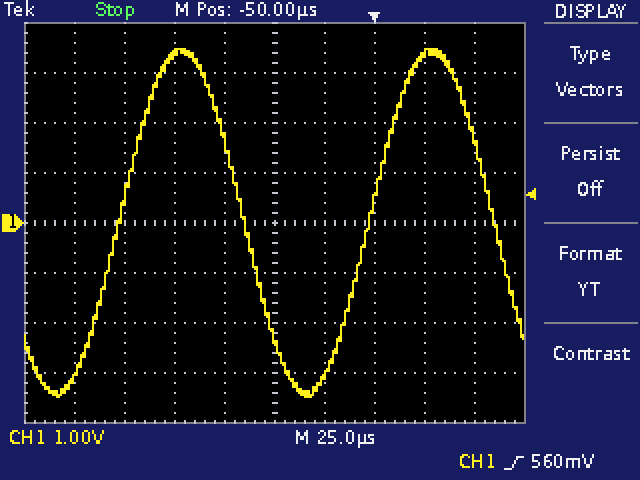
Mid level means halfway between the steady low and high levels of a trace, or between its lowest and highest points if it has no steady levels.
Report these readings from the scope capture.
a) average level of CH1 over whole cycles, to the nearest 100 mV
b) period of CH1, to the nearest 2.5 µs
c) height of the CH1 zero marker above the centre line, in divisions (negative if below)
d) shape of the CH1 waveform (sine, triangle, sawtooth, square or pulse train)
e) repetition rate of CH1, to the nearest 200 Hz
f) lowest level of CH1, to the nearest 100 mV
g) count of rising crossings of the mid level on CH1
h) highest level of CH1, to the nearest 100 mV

0.0 V
125.0 µs
0.0 div
sine
8.0 kHz
-3.5 V
2
3.5 V
